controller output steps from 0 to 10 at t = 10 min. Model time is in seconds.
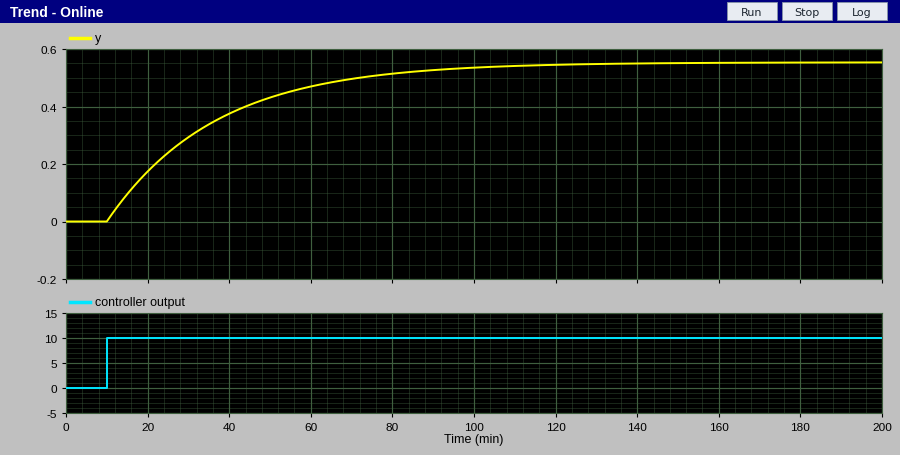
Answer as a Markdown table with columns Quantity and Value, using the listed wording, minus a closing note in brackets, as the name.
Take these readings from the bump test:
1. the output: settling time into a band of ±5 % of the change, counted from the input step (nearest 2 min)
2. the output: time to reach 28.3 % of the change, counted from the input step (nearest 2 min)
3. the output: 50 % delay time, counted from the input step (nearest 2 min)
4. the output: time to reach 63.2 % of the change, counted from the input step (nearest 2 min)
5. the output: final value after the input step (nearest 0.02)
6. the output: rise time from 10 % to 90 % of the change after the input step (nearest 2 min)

| Quantity | Value |
|---|---|
| the output: settling time into a band of ±5 % of the change, counted from the input step | 80 min |
| the output: time to reach 28.3 % of the change, counted from the input step | 8 min |
| the output: 50 % delay time, counted from the input step | 18 min |
| the output: time to reach 63.2 % of the change, counted from the input step | 26 min |
| the output: final value after the input step | 0.56 |
| the output: rise time from 10 % to 90 % of the change after the input step | 58 min |
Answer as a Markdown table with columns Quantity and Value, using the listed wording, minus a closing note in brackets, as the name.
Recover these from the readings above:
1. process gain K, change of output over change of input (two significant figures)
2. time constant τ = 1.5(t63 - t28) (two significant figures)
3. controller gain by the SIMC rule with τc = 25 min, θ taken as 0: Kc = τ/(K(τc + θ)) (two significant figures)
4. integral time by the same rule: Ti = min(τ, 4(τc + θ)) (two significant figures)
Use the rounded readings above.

| Quantity | Value |
|---|---|
| process gain K, change of output over change of input | 0.056 |
| time constant τ = 1.5(t63 - t28) | 27 min |
| controller gain by the SIMC rule with τc = 25 min, θ taken as 0: Kc = τ/(K(τc + θ)) | 19 |
| integral time by the same rule: Ti = min(τ, 4(τc + θ)) | 27 min |
